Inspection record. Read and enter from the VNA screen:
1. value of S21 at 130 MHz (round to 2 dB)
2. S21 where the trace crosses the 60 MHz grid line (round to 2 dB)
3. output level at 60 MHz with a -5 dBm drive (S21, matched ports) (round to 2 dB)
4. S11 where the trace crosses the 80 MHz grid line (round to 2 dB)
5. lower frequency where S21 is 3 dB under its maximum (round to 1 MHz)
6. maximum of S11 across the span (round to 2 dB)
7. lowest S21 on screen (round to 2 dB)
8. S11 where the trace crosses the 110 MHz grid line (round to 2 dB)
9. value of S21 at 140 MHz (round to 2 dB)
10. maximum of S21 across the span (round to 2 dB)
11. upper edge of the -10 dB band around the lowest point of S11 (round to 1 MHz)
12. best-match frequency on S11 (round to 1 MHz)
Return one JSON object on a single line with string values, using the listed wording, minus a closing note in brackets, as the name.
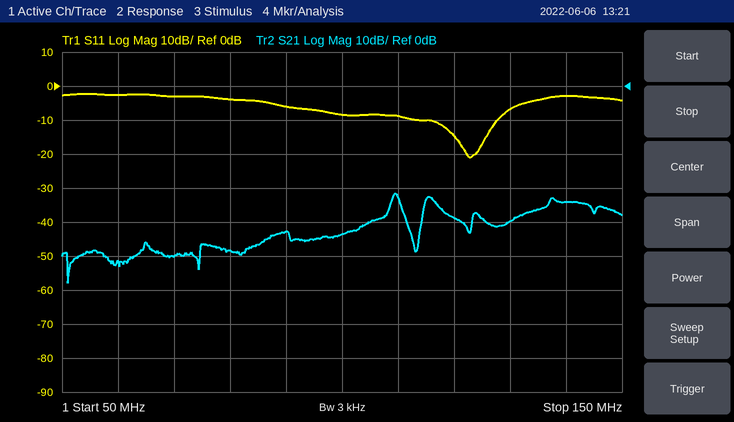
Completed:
{"value of S21 at 130 MHz": "-40 dB", "S21 where the trace crosses the 60 MHz grid line": "-52 dB", "output level at 60 MHz with a -5 dBm drive (S21, matched ports)": "-56 dBm", "S11 where the trace crosses the 80 MHz grid line": "-4 dB", "lower frequency where S21 is 3 dB under its maximum": "109 MHz", "maximum of S11 across the span": "-2 dB", "lowest S21 on screen": "-58 dB", "S11 where the trace crosses the 110 MHz grid line": "-8 dB", "value of S21 at 140 MHz": "-34 dB", "maximum of S21 across the span": "-32 dB", "upper edge of the -10 dB band around the lowest point of S11": "128 MHz", "best-match frequency on S11": "123 MHz"}
